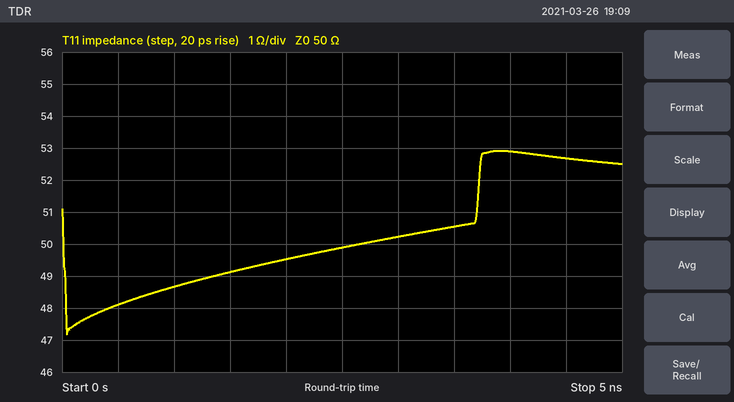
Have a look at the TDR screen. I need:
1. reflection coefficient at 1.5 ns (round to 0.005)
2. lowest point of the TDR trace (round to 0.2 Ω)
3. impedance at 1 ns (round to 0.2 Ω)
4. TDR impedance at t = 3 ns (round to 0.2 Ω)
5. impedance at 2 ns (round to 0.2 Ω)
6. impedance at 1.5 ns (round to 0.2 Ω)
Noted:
-0.010
47.2 Ω
48.6 Ω
50.2 Ω
49.6 Ω
49.2 Ω
